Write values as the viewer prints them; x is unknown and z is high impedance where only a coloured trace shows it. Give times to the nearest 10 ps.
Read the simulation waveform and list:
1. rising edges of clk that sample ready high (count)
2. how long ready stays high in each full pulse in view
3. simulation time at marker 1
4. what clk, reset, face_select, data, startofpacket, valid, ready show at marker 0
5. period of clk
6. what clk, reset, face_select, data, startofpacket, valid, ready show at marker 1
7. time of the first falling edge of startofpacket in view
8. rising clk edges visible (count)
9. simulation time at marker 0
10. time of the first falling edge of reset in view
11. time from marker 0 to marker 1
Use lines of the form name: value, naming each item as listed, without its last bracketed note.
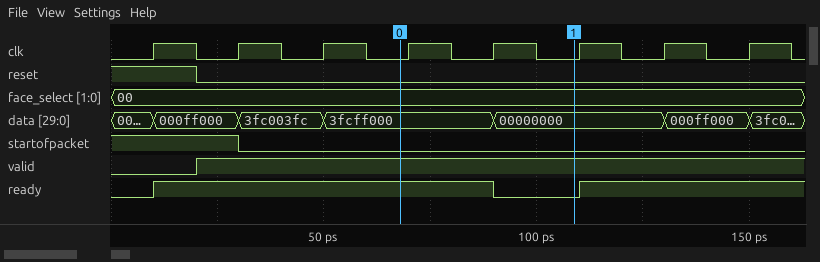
rising edges of clk that sample ready high: 6
how long ready stays high in each full pulse in view: 80 ps
simulation time at marker 1: 110 ps
what clk, reset, face_select, data, startofpacket, valid, ready show at marker 0: clk=0, reset=0, face_select=00, data=3fcff000, startofpacket=0, valid=1, ready=1
period of clk: 20 ps
what clk, reset, face_select, data, startofpacket, valid, ready show at marker 1: clk=0, reset=0, face_select=00, data=00000000, startofpacket=0, valid=1, ready=0
time of the first falling edge of startofpacket in view: 30 ps
rising clk edges visible: 8
simulation time at marker 0: 70 ps
time of the first falling edge of reset in view: 20 ps
time from marker 0 to marker 1: 40 ps
